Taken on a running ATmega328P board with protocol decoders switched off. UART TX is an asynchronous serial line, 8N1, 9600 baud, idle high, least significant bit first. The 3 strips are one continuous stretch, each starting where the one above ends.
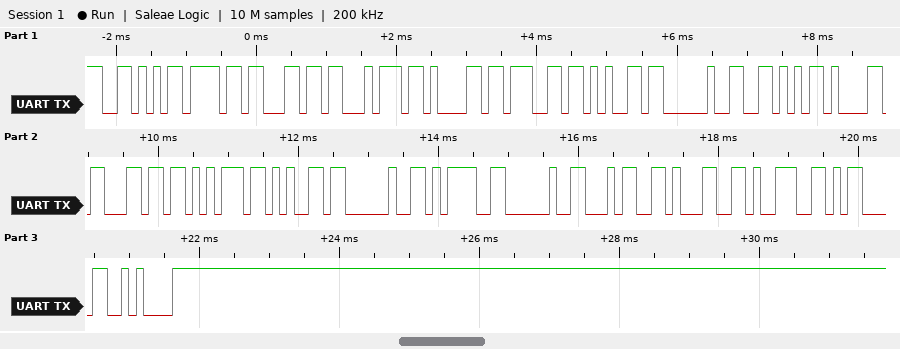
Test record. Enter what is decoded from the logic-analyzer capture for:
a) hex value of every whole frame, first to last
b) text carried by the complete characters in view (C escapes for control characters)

0x56 0x6F 0x6C 0x74 0x61 0x67 0x65 0x20 0x56 0x61 0x6C 0x75 0x65 0x20 0x3D 0x20 0x34 0x31 0x39 0x0D 0x0A
"Voltage Value = 419\r\n"
